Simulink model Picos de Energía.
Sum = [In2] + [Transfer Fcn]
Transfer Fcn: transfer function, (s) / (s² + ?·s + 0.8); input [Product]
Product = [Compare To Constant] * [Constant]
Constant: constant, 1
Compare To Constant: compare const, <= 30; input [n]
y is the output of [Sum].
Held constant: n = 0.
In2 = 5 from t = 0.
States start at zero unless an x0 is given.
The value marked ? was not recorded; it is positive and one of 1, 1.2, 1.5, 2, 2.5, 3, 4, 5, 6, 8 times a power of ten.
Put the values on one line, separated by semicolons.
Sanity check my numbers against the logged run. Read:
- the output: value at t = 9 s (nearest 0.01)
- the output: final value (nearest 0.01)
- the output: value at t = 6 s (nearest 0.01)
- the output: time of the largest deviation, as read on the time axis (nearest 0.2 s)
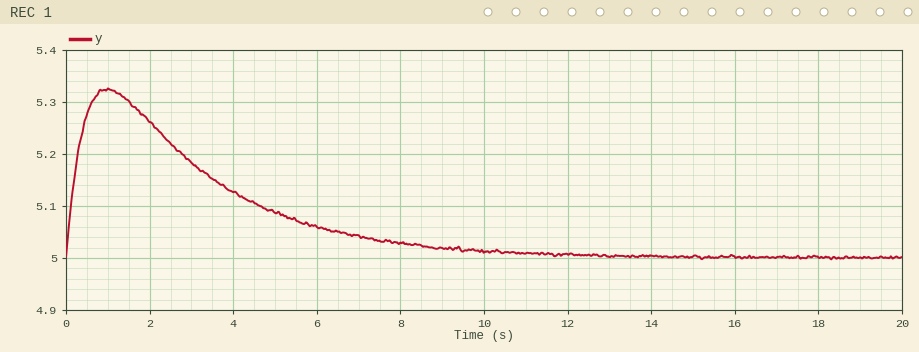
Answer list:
5.02; 5.00; 5.06; 1.0 s
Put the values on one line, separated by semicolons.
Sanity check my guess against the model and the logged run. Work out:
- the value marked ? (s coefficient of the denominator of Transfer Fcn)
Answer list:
2.5
